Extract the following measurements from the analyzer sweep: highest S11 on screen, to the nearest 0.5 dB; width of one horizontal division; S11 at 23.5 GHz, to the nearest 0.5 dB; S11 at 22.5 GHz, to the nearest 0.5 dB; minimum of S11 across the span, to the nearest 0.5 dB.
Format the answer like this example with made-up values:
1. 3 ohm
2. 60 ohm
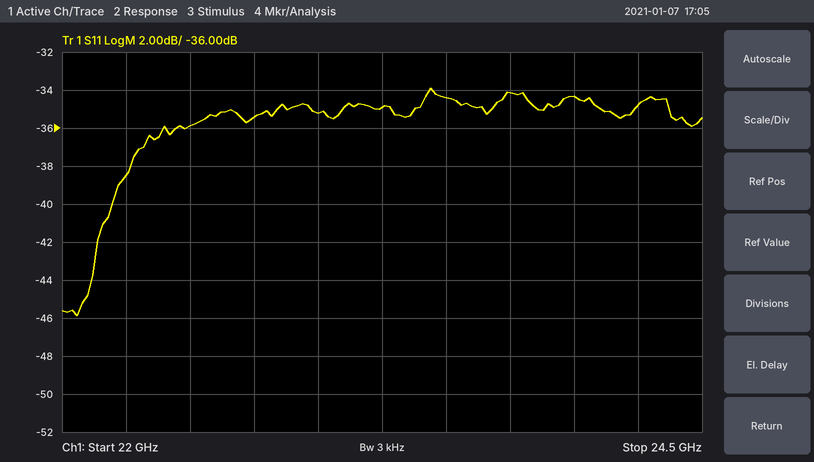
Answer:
1. -34.0 dB
2. 250 MHz
3. -34.5 dB
4. -36.0 dB
5. -46.0 dB
